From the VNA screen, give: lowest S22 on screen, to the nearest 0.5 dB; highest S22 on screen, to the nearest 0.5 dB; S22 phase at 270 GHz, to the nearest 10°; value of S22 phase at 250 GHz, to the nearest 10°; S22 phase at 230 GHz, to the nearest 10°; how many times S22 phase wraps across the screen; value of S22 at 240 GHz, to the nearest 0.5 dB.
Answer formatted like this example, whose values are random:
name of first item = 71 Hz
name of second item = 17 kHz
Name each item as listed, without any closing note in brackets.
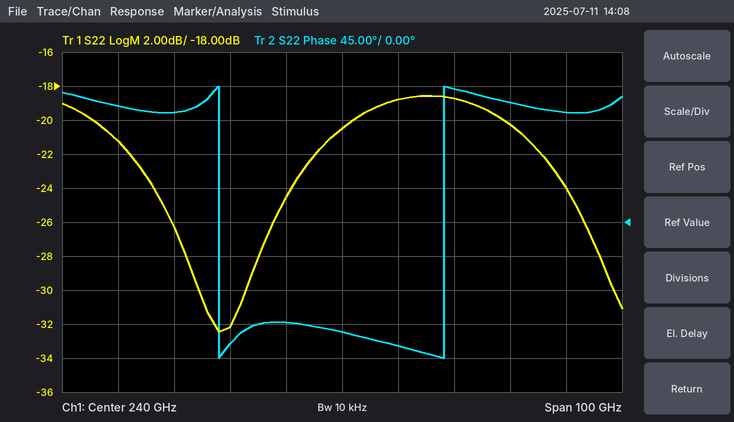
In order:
lowest S22 on screen, to the nearest 0.5 dB = -32.5 dB
highest S22 on screen, to the nearest 0.5 dB = -18.5 dB
S22 phase at 270 GHz, to the nearest 10° = 160°
value of S22 phase at 250 GHz, to the nearest 10° = -160°
S22 phase at 230 GHz, to the nearest 10° = -130°
how many times S22 phase wraps across the screen = 2
value of S22 at 240 GHz, to the nearest 0.5 dB = -20.5 dB
